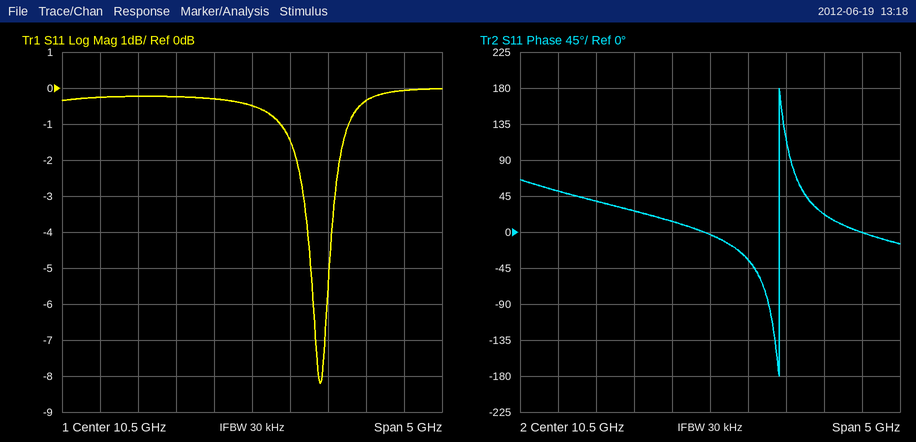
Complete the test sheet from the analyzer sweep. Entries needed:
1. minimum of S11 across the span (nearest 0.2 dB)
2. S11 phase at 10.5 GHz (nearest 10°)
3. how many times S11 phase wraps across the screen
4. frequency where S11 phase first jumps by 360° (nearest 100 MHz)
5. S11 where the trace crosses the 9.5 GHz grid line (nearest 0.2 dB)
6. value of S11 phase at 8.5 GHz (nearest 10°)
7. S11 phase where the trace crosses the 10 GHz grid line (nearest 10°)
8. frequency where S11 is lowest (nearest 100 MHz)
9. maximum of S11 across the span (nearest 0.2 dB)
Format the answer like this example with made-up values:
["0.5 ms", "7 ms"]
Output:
["-8.2 dB", "0°", "1", "11.4 GHz", "-0.2 dB", "50°", "10°", "11.4 GHz", "0.0 dB"]
